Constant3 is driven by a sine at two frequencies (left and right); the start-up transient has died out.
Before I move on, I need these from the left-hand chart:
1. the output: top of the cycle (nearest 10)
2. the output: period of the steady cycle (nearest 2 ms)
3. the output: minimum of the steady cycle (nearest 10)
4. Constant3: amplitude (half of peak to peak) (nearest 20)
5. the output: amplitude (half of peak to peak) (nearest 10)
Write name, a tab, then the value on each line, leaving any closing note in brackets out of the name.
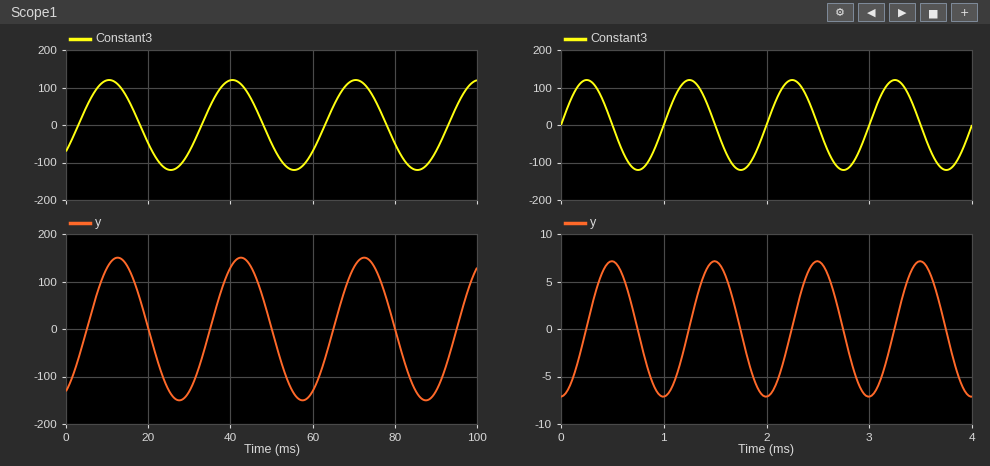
the output: top of the cycle	150
the output: period of the steady cycle	30 ms
the output: minimum of the steady cycle	-150
Constant3: amplitude (half of peak to peak)	120
the output: amplitude (half of peak to peak)	150
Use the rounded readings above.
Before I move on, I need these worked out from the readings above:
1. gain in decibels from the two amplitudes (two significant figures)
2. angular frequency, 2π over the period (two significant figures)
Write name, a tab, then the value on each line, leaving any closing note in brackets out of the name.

gain in decibels from the two amplitudes	1.9 dB
angular frequency, 2π over the period	0.21 rad/ms
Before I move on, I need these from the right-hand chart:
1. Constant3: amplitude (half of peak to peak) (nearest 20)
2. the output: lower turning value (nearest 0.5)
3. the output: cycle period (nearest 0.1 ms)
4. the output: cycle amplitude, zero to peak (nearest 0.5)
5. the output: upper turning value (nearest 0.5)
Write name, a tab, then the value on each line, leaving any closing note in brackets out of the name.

Constant3: amplitude (half of peak to peak)	120
the output: lower turning value	-7.0
the output: cycle period	1.0 ms
the output: cycle amplitude, zero to peak	7.0
the output: upper turning value	7.0
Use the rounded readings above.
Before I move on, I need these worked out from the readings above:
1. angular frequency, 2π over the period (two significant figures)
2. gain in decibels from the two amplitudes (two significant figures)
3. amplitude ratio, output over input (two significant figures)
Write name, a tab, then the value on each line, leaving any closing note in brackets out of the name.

angular frequency, 2π over the period	6.3 rad/ms
gain in decibels from the two amplitudes	-25 dB
amplitude ratio, output over input	0.058
